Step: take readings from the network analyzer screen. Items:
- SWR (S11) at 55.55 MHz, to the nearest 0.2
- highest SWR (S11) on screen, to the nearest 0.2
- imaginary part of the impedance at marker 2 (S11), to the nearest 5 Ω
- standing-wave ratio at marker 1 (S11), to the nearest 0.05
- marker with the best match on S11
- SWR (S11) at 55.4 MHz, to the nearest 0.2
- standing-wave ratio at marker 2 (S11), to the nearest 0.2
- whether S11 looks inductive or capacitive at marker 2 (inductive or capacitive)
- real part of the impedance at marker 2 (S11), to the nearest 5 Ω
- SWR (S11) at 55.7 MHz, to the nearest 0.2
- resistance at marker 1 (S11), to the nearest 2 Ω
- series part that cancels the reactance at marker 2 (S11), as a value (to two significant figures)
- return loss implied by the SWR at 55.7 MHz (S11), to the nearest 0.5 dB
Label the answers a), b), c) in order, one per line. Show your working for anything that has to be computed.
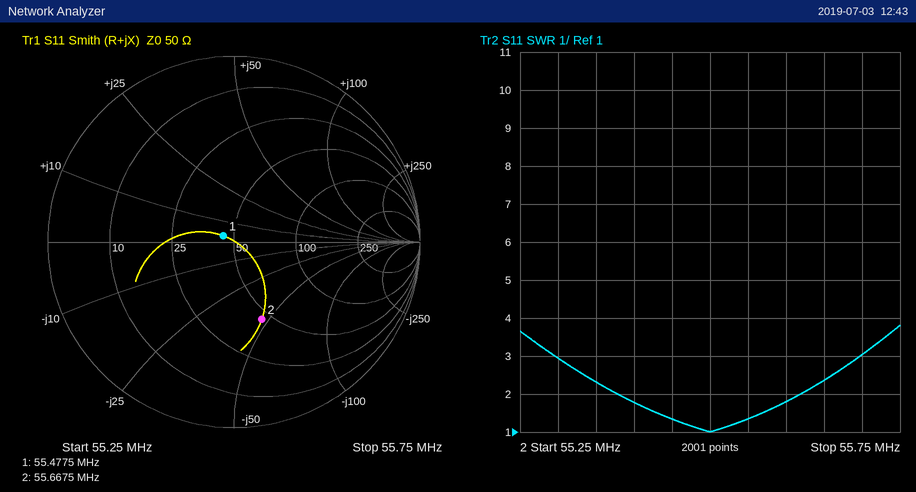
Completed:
a) 1.4
b) 3.8
c) -45 Ω
d) 1.15
e) marker 1
f) 1.8
g) 2.6
h) capacitive
i) 45 Ω
j) 3.0
k) 44 Ω
l) L = 45 Ω/(2π × 55.6675 MHz) ≈ 129 nH, so 130 nH to two significant figures
m) −20 log10((3 − 1)/(3 + 1)) ≈ 6.0 dB
